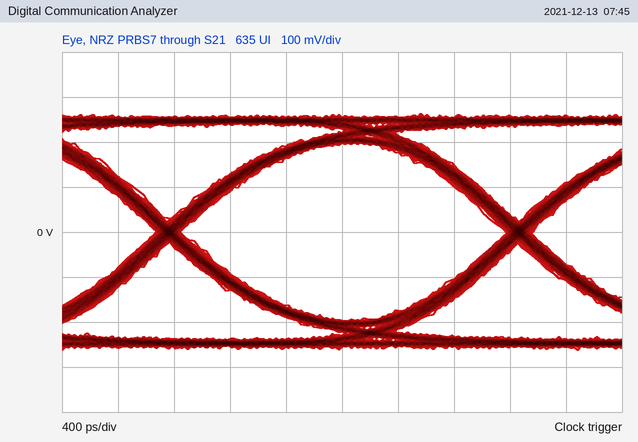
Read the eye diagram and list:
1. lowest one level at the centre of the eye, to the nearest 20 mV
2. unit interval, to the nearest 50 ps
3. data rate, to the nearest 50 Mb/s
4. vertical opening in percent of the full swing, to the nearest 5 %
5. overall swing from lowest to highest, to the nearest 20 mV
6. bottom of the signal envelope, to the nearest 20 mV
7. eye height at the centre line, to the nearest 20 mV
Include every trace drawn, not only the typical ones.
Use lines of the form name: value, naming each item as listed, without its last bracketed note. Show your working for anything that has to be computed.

lowest one level at the centre of the eye, to the nearest 20 mV: 200 mV
unit interval, to the nearest 50 ps: 2.50 ns
data rate, to the nearest 50 Mb/s: 400 Mb/s
vertical opening in percent of the full swing, to the nearest 5 %: 400 mV / 520 mV ≈ 76.9 %, so 75 % to the nearest 5 %
overall swing from lowest to highest, to the nearest 20 mV: 520 mV
bottom of the signal envelope, to the nearest 20 mV: -260 mV
eye height at the centre line, to the nearest 20 mV: 400 mV
